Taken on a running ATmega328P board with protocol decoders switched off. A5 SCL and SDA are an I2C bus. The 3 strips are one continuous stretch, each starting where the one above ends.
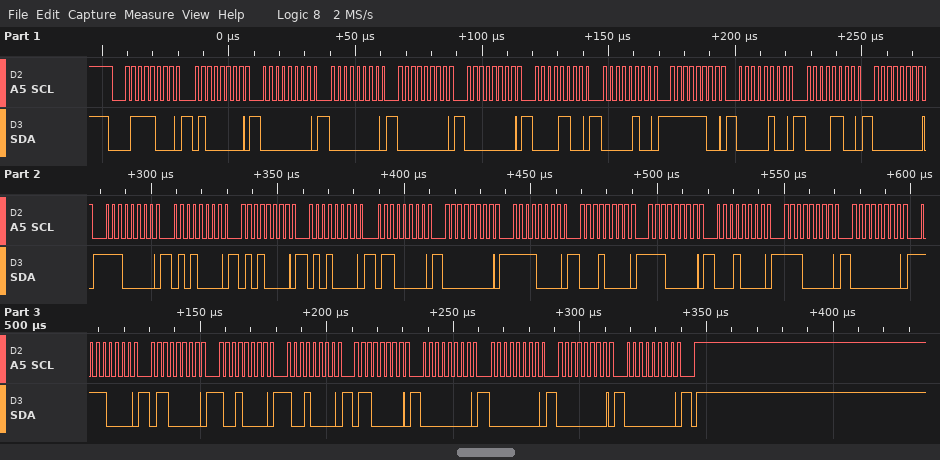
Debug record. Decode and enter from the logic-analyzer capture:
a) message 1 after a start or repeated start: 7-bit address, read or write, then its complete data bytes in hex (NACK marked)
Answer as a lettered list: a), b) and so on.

a) 0x3C write: 40 00 00 00 00 0C 04 FC 04 0C 00 E0 50 50 50 60 00 F0 10 E0 10 E0 00 F0 60 90 90 60 00 00 00 00
